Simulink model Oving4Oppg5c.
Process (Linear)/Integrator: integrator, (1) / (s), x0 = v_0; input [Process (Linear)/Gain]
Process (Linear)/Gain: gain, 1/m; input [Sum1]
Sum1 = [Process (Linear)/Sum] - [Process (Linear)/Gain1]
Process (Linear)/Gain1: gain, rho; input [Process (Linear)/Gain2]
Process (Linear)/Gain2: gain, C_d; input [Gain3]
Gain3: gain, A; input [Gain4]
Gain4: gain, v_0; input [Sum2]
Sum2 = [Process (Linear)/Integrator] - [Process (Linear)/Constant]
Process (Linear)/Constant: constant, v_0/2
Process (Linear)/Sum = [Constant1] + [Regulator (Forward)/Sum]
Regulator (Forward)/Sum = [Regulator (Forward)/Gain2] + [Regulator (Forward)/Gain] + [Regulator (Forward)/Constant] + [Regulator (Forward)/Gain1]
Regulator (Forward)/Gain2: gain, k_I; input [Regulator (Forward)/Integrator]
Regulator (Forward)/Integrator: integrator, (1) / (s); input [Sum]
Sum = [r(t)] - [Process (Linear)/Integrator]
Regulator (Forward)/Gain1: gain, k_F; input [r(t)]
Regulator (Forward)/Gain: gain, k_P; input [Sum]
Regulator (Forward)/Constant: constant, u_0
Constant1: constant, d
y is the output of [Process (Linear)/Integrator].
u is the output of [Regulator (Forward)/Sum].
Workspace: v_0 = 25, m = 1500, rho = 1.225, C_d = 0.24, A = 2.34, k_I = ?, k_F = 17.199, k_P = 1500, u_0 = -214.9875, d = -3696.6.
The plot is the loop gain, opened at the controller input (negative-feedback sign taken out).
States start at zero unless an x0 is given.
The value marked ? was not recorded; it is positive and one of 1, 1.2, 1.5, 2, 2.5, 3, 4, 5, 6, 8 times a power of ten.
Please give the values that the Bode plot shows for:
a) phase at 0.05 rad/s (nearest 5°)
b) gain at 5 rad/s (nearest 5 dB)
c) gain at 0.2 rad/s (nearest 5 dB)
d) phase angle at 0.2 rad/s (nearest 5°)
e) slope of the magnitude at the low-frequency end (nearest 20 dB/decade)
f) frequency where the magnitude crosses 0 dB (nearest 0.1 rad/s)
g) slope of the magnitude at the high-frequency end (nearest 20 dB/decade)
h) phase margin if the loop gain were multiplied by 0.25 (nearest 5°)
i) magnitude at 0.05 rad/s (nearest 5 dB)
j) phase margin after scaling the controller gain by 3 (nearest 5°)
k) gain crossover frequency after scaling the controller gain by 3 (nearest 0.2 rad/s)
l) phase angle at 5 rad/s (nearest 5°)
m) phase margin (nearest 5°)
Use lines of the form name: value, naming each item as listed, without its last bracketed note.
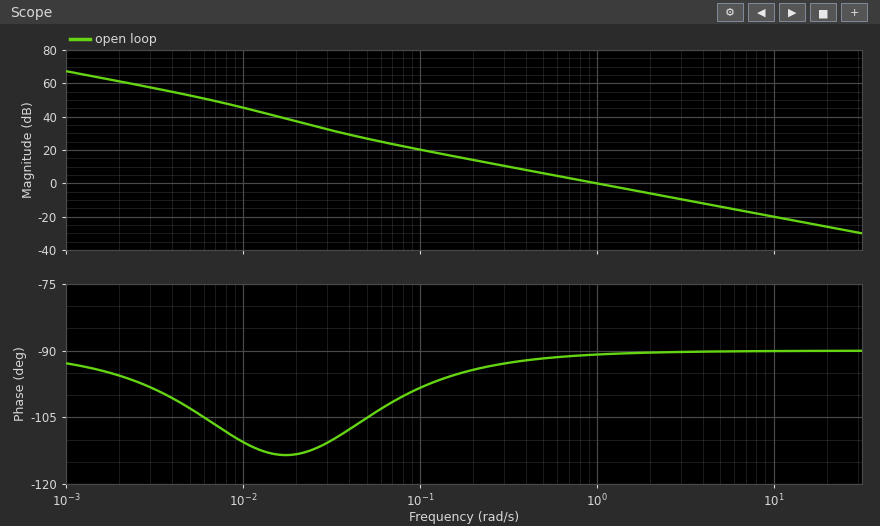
phase at 0.05 rad/s: -105°
gain at 5 rad/s: -15 dB
gain at 0.2 rad/s: 15 dB
phase angle at 0.2 rad/s: -95°
slope of the magnitude at the low-frequency end: -20 dB/decade
frequency where the magnitude crosses 0 dB: 1.0 rad/s
slope of the magnitude at the high-frequency end: -20 dB/decade
phase margin if the loop gain were multiplied by 0.25: 85°
magnitude at 0.05 rad/s: 25 dB
phase margin after scaling the controller gain by 3: 90°
gain crossover frequency after scaling the controller gain by 3: 3.0 rad/s
phase angle at 5 rad/s: -90°
phase margin: 90°
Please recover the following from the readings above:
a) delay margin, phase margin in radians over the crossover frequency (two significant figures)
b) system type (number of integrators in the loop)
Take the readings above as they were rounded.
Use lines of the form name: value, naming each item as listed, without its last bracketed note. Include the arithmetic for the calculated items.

delay margin, phase margin in radians over the crossover frequency: 90 × π / 180 / 1 = 1.6 s
system type: 1
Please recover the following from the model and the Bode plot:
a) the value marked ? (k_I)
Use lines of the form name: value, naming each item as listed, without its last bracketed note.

the value marked ?: 40
